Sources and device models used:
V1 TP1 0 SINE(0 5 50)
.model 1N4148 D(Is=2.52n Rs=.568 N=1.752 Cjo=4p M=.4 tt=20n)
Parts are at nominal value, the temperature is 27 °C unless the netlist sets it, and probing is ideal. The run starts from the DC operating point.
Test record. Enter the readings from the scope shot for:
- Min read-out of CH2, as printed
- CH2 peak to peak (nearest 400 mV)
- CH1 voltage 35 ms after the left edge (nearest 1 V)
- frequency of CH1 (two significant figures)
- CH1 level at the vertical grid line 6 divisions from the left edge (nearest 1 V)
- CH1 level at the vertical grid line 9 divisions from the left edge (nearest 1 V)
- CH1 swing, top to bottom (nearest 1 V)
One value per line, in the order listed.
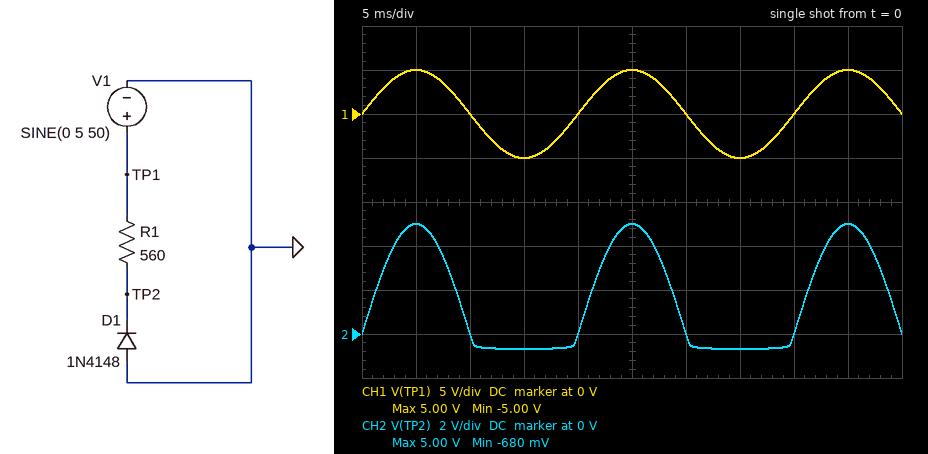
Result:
-680 mV
5.6 V
-5 V
50 Hz
0 V
5 V
10 V
